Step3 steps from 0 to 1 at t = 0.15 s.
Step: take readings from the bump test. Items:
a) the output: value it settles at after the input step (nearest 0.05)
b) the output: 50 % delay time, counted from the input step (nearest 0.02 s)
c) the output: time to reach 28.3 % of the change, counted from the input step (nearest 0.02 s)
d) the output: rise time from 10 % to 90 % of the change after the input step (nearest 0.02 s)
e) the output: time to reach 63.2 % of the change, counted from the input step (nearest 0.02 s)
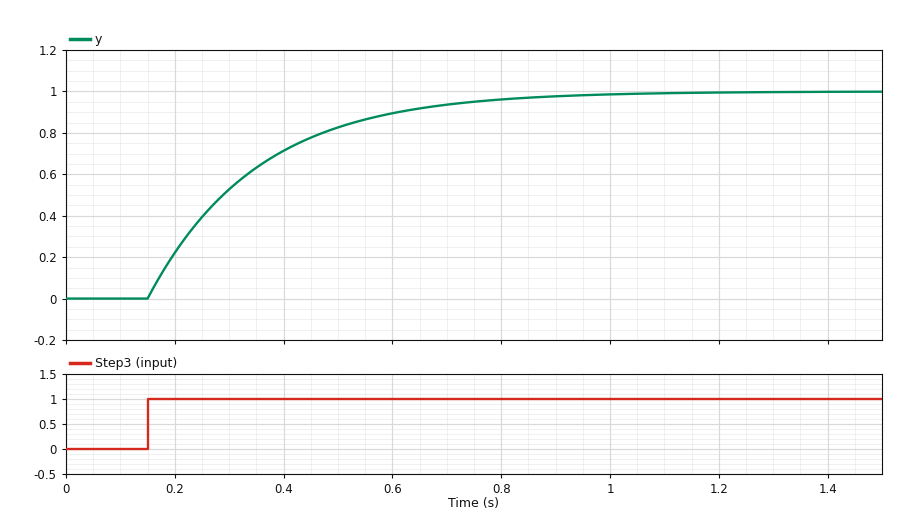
1.00
0.14 s
0.06 s
0.44 s
0.20 s
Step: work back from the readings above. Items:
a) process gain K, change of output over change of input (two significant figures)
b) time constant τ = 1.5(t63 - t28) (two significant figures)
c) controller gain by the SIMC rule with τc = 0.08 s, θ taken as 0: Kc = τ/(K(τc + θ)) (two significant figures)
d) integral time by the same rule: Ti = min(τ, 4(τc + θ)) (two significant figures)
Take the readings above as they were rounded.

1.0
0.21 s
2.6
0.21 s
